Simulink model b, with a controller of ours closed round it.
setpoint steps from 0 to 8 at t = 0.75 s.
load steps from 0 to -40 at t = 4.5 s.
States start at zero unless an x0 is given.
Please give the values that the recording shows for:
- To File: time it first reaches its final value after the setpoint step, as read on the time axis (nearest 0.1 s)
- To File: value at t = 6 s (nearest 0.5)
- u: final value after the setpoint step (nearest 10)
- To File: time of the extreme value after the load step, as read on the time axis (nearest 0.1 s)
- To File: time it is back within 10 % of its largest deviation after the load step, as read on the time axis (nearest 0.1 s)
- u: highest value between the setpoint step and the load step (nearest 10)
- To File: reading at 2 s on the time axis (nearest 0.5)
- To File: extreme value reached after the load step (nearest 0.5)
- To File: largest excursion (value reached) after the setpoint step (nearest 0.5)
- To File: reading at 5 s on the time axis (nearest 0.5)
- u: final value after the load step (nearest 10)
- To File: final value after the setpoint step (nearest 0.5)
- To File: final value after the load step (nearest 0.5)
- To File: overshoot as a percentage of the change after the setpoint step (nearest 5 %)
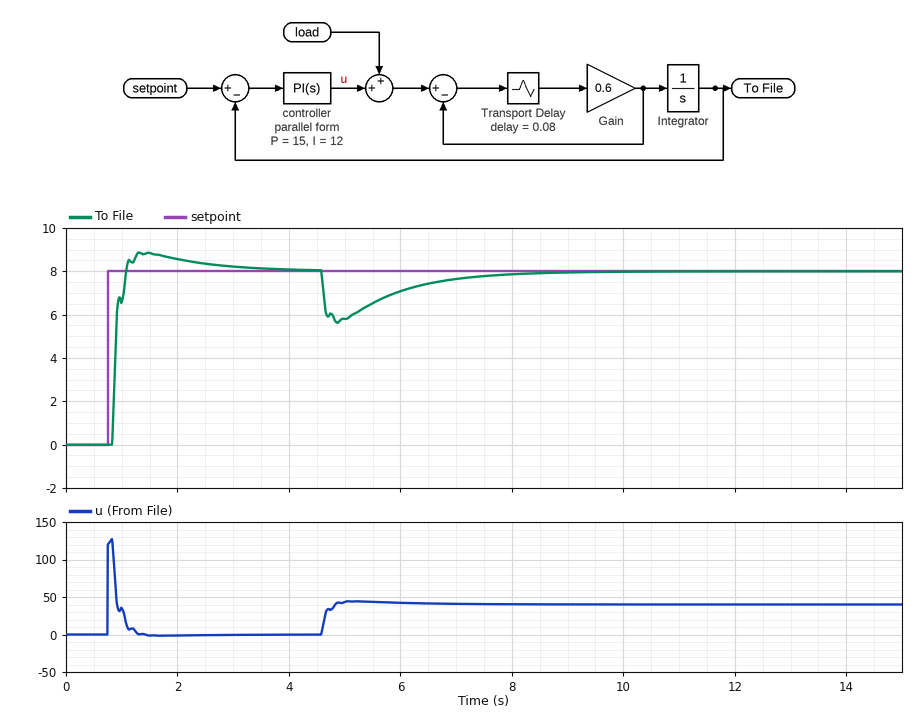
1.1 s
7.0
0
4.9 s
7.4 s
130
8.5
5.5
9.0
6.0
40
8.0
8.0
10 %
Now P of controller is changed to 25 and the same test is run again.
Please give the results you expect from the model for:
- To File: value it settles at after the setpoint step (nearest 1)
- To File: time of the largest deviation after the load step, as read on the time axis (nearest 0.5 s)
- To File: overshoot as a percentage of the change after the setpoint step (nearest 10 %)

8
4.5 s
30 %
